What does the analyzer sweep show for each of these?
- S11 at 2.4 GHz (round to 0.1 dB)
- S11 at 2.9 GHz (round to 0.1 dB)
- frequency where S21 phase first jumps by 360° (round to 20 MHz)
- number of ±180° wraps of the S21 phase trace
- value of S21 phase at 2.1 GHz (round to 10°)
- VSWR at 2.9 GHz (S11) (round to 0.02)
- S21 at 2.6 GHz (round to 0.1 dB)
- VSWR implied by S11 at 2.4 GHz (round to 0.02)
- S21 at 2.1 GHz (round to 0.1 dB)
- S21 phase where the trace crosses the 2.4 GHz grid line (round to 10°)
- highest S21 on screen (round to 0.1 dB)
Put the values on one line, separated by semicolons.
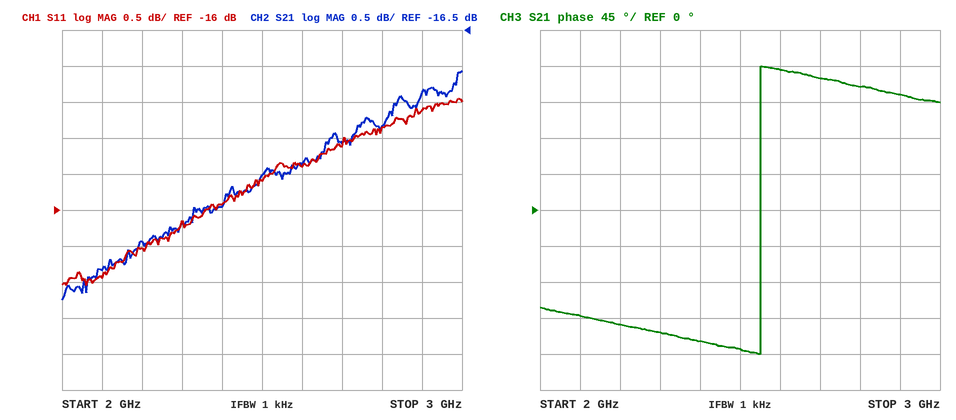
-15.9 dB; -14.6 dB; 2.56 GHz; 1; -130°; 1.46; -18.4 dB; 1.38; -19.8 dB; -160°; -17.1 dB
